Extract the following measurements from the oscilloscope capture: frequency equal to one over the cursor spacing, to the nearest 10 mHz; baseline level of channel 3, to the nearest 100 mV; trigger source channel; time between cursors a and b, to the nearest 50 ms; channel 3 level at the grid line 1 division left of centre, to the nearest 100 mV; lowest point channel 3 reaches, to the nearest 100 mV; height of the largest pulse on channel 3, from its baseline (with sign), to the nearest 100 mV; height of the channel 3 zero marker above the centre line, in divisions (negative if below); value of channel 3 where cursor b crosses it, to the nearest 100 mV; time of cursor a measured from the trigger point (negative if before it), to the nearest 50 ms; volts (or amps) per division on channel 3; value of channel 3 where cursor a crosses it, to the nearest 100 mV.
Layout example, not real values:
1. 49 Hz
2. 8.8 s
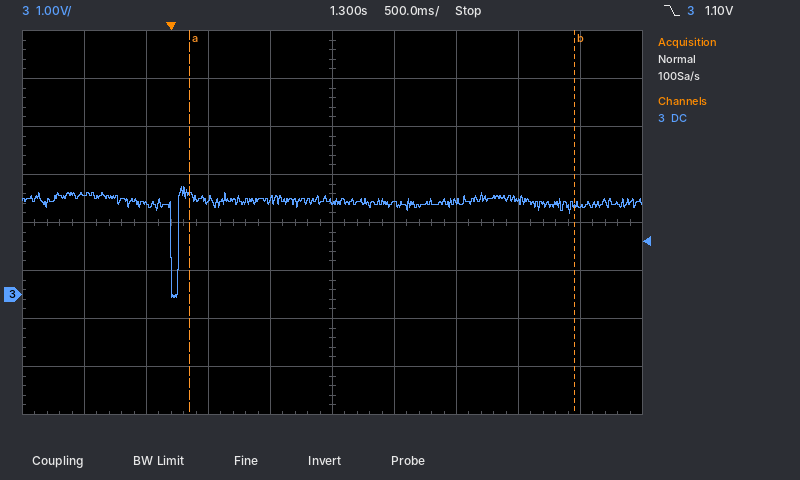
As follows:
1. 320 mHz
2. 1.9 V
3. channel 3
4. 3.10 s
5. 2.0 V
6. -100 mV
7. -2.0 V
8. -1.5 div
9. 1.9 V
10. +150 ms
11. 1 V
12. 2.1 V
